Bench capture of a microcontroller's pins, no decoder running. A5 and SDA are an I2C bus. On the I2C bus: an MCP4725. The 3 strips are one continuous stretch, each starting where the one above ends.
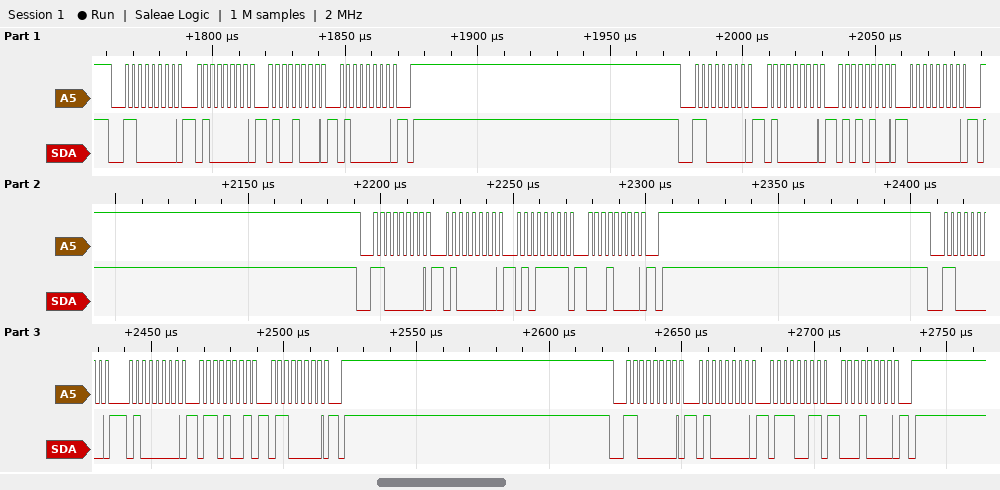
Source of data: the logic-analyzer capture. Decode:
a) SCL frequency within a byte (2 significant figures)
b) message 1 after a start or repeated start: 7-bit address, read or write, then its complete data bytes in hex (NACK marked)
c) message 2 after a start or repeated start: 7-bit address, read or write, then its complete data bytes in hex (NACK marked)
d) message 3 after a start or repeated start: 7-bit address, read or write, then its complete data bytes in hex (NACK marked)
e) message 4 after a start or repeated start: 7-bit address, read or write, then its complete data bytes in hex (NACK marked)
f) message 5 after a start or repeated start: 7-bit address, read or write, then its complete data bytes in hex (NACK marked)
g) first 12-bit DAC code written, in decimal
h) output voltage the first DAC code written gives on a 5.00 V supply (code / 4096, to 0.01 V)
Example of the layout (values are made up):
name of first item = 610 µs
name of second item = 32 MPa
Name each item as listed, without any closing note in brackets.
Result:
SCL frequency within a byte = 400 kHz
message 1 after a start or repeated start: 7-bit address, read or write, then its complete data bytes in hex = 0x60 write: 40 48 40
message 2 after a start or repeated start: 7-bit address, read or write, then its complete data bytes in hex = 0x60 write: 40 54 00
message 3 after a start or repeated start: 7-bit address, read or write, then its complete data bytes in hex = 0x60 write: 40 5F 10
message 4 after a start or repeated start: 7-bit address, read or write, then its complete data bytes in hex = 0x60 write: 40 69 60
message 5 after a start or repeated start: 7-bit address, read or write, then its complete data bytes in hex = 0x60 write: 40 73 10
first 12-bit DAC code written, in decimal = 1156
output voltage the first DAC code written gives on a 5.00 V supply = 1.41 V
